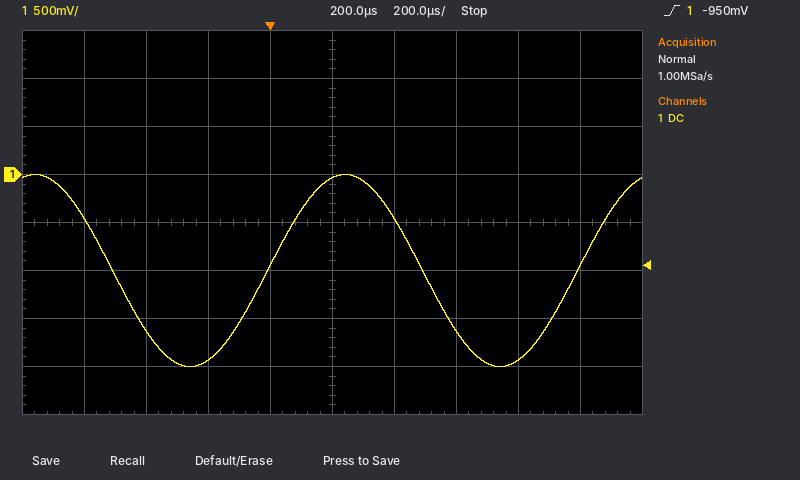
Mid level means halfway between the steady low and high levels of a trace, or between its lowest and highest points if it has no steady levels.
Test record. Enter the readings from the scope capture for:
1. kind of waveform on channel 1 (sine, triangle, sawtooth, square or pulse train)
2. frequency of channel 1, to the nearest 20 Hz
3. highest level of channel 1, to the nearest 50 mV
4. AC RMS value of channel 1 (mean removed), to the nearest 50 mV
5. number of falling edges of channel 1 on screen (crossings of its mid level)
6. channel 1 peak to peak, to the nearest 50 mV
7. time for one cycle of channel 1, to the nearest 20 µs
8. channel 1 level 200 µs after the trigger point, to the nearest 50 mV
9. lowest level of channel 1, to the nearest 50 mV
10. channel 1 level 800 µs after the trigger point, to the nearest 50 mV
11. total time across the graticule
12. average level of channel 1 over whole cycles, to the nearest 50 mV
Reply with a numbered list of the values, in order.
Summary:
1. sine
2. 1.00 kHz
3. 0 mV
4. 700 mV
5. 2
6. 2.00 V
7. 1.00 ms
8. -50 mV
9. -2.00 V
10. -1.95 V
11. 2 ms
12. -1.00 V
